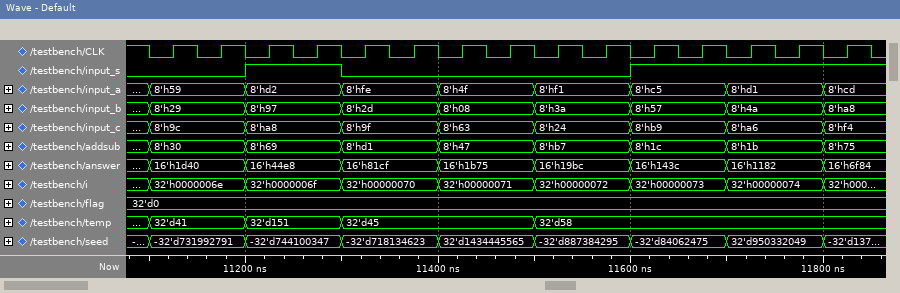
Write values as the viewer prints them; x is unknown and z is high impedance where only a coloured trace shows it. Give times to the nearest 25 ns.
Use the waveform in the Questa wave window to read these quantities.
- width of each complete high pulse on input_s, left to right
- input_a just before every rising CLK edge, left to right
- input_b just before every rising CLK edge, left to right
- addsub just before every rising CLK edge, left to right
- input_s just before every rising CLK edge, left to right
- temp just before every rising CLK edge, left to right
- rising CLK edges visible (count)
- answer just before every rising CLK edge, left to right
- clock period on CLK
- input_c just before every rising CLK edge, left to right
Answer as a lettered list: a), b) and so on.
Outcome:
a) 100 ns
b) 8'h59, 8'h59, 8'hd2, 8'hd2, 8'hfe, 8'hfe, 8'h4f, 8'h4f, 8'hf1, 8'hf1, 8'hc5, 8'hc5, 8'hd1, 8'hd1, 8'hcd
c) 8'h29, 8'h29, 8'h97, 8'h97, 8'h2d, 8'h2d, 8'h08, 8'h08, 8'h3a, 8'h3a, 8'h57, 8'h57, 8'h4a, 8'h4a, 8'ha8
d) 8'h30, 8'h30, 8'h69, 8'h69, 8'hd1, 8'hd1, 8'h47, 8'h47, 8'hb7, 8'hb7, 8'h1c, 8'h1c, 8'h1b, 8'h1b, 8'h75
e) 0 0 1 1 0 0 0 0 0 0 1 1 1 1 1
f) 32'd41, 32'd41, 32'd151, 32'd151, 32'd45, 32'd45, 32'd45, 32'd45, 32'd58, 32'd58, 32'd58, 32'd58, 32'd58, 32'd58, 32'd58
g) 15
h) 16'h1d40, 16'h1d40, 16'h44e8, 16'h44e8, 16'h81cf, 16'h81cf, 16'h1b75, 16'h1b75, 16'h19bc, 16'h19bc, 16'h143c, 16'h143c, 16'h1182, 16'h1182, 16'h6f84
i) 50 ns
j) 8'h9c, 8'h9c, 8'ha8, 8'ha8, 8'h9f, 8'h9f, 8'h63, 8'h63, 8'h24, 8'h24, 8'hb9, 8'hb9, 8'ha6, 8'ha6, 8'hf4
